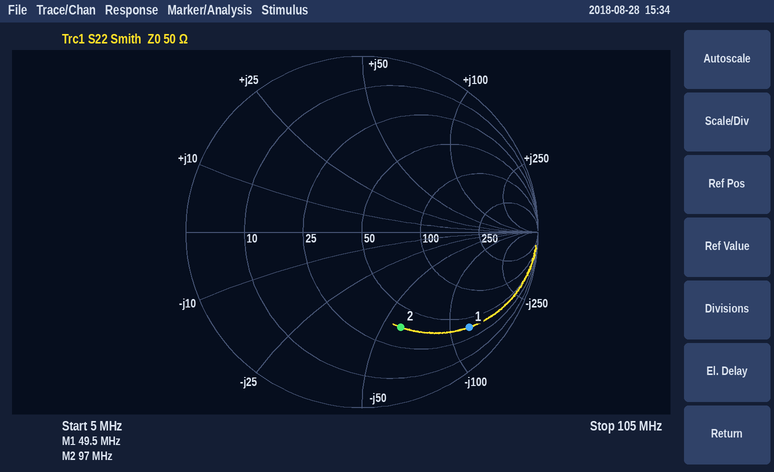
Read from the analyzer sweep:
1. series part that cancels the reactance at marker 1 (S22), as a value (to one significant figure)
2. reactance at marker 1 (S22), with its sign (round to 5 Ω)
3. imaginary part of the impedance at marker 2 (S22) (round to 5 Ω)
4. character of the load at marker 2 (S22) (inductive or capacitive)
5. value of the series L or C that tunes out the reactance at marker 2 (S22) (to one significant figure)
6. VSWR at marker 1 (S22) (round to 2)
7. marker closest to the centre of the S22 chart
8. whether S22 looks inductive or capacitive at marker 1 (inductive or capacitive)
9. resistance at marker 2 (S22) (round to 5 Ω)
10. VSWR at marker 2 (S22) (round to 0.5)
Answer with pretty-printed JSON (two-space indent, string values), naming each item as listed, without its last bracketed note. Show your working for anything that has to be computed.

{
  "series part that cancels the reactance at marker 1 (S22), as a value": "L = 120 Ω/(2π × 49.5 MHz) ≈ 386 nH, so 400 nH to one significant figure",
  "reactance at marker 1 (S22), with its sign": "-120 Ω",
  "imaginary part of the impedance at marker 2 (S22)": "-60 Ω",
  "character of the load at marker 2 (S22)": "capacitive",
  "value of the series L or C that tunes out the reactance at marker 2 (S22)": "L = 60 Ω/(2π × 97 MHz) ≈ 98.4 nH, so 100 nH to one significant figure",
  "VSWR at marker 1 (S22)": "10",
  "marker closest to the centre of the S22 chart": "marker 2",
  "whether S22 looks inductive or capacitive at marker 1": "capacitive",
  "resistance at marker 2 (S22)": "35 Ω",
  "VSWR at marker 2 (S22)": "4.0"
}
